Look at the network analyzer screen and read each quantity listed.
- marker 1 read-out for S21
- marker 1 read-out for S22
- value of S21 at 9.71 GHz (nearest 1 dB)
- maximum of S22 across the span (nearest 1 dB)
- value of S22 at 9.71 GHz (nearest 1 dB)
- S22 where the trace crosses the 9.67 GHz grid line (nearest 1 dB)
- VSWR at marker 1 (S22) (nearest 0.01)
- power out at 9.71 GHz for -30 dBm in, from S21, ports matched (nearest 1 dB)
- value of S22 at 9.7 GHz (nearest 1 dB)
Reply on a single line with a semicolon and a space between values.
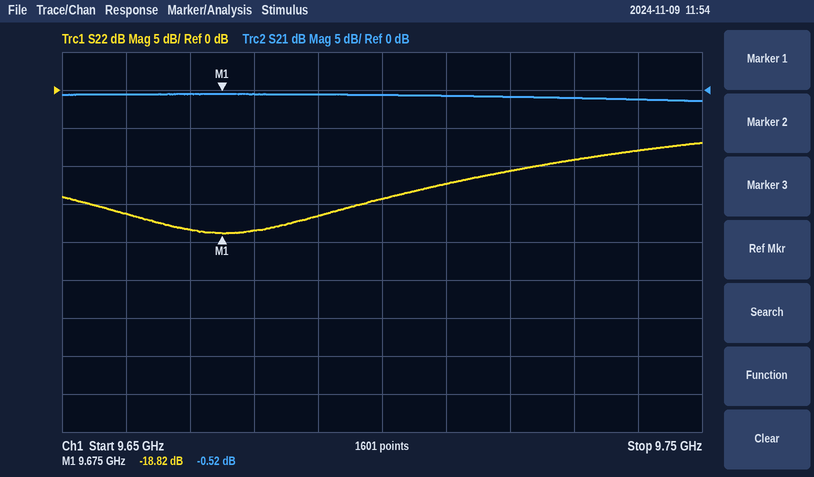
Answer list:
-0.52 dB; -18.82 dB; -1 dB; -7 dB; -12 dB; -18 dB; 1.26; -31 dBm; -14 dB
